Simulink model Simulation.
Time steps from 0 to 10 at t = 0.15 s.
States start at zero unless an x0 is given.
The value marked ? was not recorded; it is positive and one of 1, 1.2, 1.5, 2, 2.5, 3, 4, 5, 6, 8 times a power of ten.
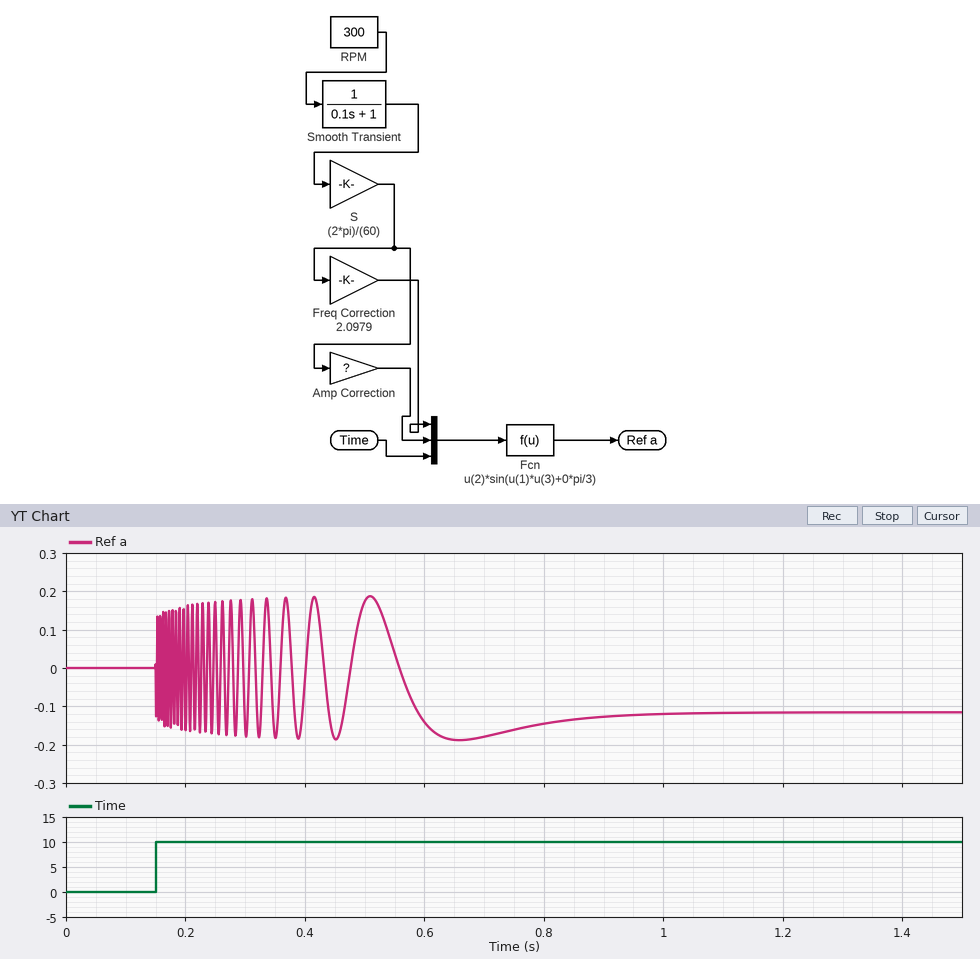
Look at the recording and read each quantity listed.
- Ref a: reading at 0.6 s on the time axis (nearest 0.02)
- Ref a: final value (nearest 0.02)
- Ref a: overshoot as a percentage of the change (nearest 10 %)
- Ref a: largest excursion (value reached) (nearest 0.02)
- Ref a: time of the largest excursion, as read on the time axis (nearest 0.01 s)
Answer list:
-0.14
-0.12
60 %
-0.18
0.66 s
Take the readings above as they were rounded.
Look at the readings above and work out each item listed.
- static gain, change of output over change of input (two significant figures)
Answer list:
-0.012
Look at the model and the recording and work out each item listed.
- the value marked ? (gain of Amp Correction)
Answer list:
0.006
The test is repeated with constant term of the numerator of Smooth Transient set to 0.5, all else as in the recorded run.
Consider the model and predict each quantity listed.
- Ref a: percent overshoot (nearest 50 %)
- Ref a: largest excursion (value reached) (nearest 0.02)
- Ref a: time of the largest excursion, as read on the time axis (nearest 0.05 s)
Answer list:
200 %
0.10
0.55 s
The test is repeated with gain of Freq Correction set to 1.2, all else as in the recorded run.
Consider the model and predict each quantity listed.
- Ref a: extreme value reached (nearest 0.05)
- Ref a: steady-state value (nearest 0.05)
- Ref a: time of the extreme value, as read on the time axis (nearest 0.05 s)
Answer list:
-0.20
0.00
0.55 s
